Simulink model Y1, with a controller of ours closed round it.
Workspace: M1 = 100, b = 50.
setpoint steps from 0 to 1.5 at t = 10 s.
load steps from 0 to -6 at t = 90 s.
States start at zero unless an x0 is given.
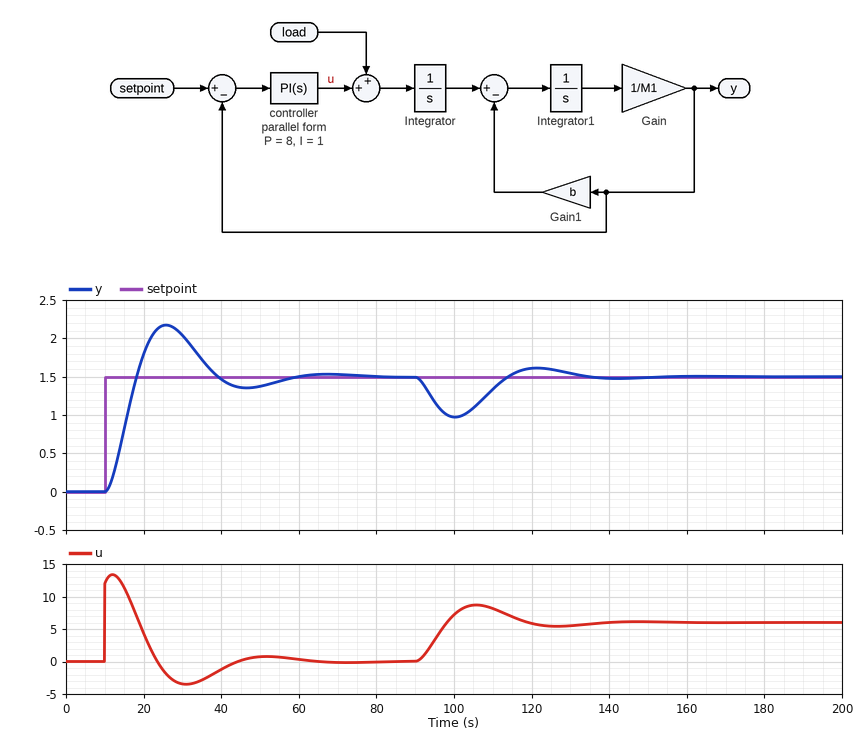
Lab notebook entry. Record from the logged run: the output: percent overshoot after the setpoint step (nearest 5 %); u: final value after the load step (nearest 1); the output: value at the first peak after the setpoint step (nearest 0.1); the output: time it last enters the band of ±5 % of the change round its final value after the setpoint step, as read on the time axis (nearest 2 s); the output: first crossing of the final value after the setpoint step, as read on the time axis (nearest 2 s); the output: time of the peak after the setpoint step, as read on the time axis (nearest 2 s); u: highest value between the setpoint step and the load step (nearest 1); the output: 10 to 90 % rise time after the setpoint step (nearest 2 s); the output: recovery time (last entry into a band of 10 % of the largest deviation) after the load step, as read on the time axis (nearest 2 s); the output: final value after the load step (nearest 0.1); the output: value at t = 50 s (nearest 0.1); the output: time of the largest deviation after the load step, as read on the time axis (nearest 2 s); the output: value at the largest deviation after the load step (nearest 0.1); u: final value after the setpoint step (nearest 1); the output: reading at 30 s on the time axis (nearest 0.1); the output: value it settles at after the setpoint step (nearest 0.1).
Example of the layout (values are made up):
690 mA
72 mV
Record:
45 %
6
2.2
54 s
18 s
26 s
13
6 s
130 s
1.5
1.4
100 s
1.0
0
2.0
1.5
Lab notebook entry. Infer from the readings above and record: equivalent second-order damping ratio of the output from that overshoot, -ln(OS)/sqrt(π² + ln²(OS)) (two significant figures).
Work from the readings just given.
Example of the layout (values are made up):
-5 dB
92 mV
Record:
0.25
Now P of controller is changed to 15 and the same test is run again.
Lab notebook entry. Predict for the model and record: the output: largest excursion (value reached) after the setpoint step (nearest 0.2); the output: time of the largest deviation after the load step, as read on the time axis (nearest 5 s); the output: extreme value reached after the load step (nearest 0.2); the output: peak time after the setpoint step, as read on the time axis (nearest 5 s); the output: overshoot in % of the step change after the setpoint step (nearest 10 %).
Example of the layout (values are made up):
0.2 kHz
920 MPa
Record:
2.0
100 s
1.2
20 s
30 %
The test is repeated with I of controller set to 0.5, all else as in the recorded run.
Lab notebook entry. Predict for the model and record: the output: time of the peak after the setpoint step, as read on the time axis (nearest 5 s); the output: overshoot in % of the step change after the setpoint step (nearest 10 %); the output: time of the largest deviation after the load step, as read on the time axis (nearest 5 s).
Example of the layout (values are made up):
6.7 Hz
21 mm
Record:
30 s
30 %
100 s
